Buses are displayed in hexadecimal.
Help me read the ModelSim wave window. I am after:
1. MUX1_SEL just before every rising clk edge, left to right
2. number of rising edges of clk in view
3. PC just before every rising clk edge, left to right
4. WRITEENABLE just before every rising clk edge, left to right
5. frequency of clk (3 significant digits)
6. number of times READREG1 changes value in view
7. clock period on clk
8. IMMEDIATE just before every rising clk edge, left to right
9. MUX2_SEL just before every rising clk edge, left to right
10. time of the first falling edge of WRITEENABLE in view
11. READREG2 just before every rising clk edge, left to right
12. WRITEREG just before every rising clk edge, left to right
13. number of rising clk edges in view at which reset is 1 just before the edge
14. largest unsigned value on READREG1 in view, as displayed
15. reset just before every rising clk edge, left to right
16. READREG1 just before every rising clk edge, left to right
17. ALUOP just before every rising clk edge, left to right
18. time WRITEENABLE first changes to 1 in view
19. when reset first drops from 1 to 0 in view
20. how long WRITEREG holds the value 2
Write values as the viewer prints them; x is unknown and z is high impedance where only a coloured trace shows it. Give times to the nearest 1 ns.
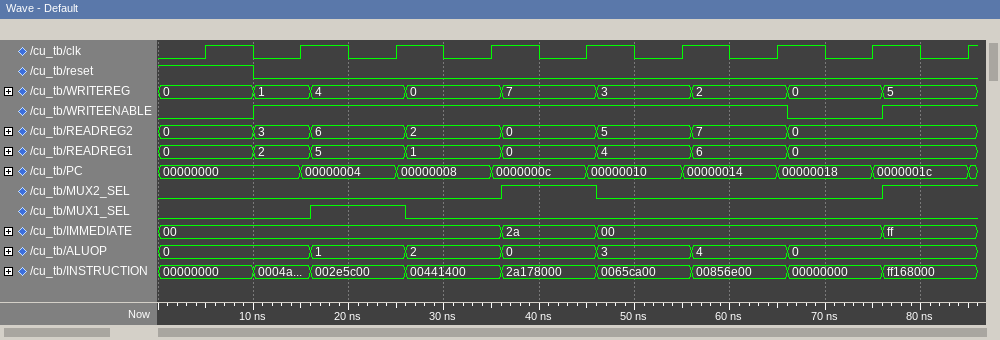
0 0 1 0 0 0 0 0 0
9
00000000, 00000000, 00000004, 00000008, 0000000c, 00000010, 00000014, 00000018, 0000001c
0 1 1 1 1 1 1 0 1
100 MHz
7
10 ns
00, 00, 00, 00, 2a, 00, 00, 00, ff
0 0 0 0 1 0 0 0 1
66 ns
0, 3, 6, 2, 0, 5, 7, 0, 0
0, 1, 4, 0, 7, 3, 2, 0, 5
1
6
1 0 0 0 0 0 0 0 0
0, 2, 5, 1, 0, 4, 6, 0, 0
0, 0, 1, 2, 0, 3, 4, 0, 0
10 ns
10 ns
10 ns
